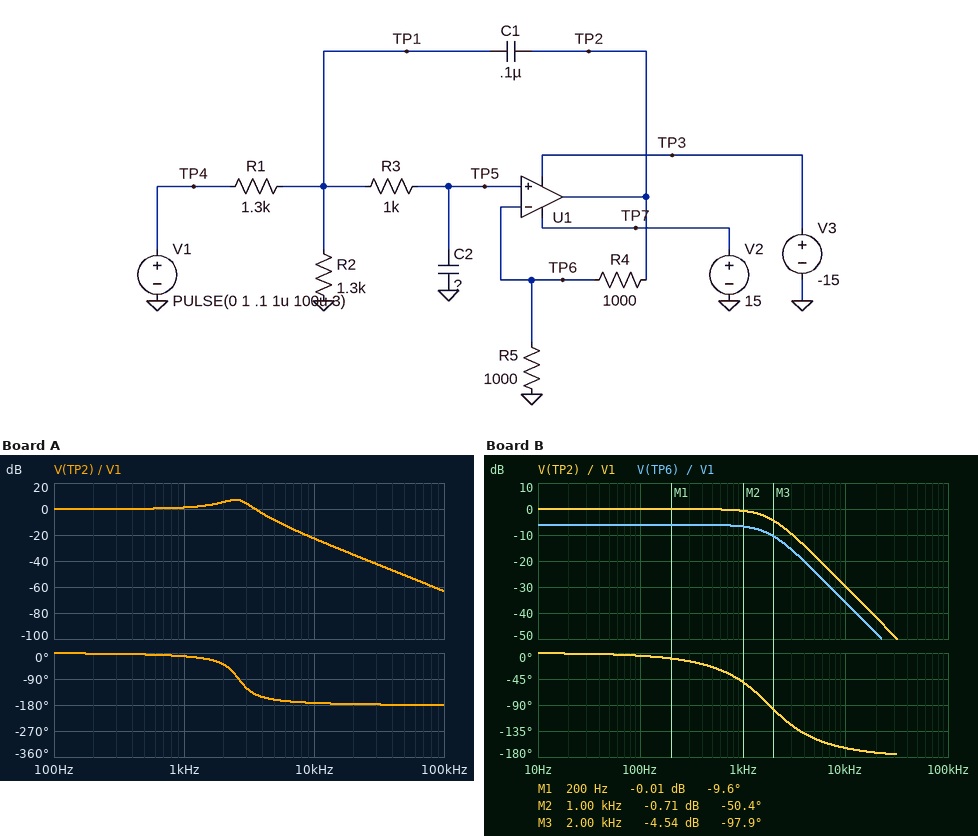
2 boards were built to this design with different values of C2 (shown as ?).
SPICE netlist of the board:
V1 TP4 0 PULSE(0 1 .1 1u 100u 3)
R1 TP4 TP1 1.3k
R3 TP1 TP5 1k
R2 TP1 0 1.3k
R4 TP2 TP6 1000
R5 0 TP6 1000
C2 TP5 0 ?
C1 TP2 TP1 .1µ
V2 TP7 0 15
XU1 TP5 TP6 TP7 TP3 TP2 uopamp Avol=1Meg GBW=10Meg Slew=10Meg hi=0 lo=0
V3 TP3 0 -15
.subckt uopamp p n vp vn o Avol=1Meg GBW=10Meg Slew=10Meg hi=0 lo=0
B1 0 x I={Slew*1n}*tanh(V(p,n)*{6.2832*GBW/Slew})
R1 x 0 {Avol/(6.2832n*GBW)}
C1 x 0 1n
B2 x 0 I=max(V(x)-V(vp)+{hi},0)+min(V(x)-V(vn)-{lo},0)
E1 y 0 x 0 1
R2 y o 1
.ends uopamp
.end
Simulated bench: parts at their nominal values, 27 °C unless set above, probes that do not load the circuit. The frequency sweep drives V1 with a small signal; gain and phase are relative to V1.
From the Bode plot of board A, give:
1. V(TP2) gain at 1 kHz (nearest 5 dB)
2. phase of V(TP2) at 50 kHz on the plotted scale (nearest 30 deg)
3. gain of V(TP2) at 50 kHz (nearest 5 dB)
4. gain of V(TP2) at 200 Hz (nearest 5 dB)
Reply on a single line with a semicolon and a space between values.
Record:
0 dB; -180 deg; -50 dB; 0 dB
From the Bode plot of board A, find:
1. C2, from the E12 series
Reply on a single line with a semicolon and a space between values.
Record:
56 nF
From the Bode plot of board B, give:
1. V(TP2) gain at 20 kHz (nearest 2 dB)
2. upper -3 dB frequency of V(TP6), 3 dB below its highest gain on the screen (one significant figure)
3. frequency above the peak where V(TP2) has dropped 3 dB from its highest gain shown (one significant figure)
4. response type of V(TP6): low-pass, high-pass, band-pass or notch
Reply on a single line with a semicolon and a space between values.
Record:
-42 dB; 2 kHz; 2 kHz; low-pass
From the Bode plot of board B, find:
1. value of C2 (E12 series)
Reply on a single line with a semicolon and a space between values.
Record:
120 nF
